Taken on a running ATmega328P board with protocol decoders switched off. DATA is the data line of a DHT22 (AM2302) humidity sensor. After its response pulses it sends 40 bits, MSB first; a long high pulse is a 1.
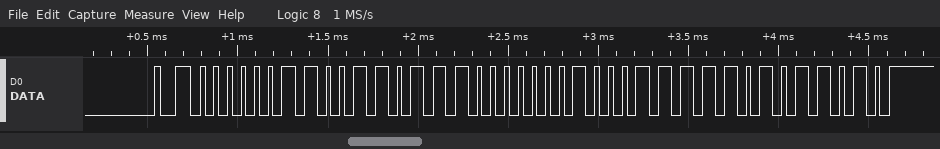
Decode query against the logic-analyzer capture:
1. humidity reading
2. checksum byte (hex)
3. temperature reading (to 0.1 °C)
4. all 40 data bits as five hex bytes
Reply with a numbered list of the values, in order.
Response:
1. 82.3 %
2. 0x5A
3. 28.7 °C
4. 03 37 01 1F 5A
